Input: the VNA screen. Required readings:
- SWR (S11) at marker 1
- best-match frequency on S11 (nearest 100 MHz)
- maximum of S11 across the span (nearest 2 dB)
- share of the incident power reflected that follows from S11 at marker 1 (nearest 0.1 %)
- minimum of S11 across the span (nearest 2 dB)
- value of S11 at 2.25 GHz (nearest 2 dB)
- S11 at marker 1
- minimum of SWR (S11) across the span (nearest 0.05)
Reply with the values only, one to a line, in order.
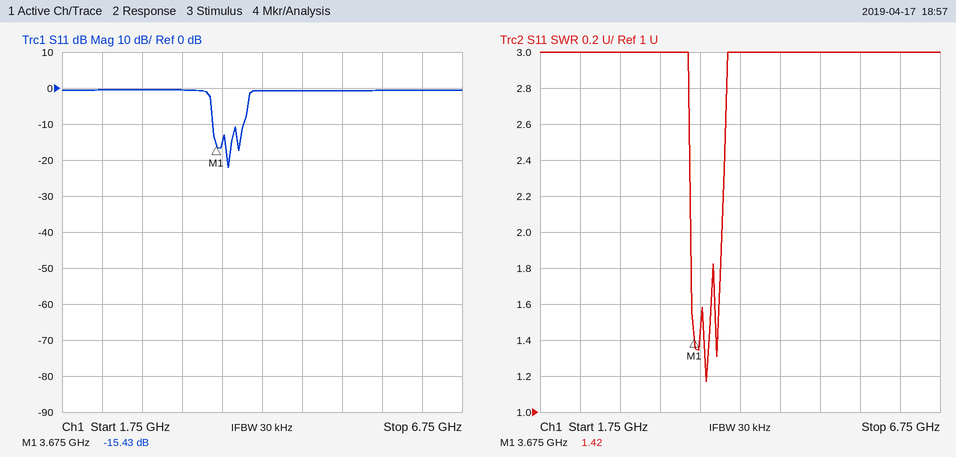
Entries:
1.42
3.8 GHz
0 dB
2.9 %
-22 dB
0 dB
-15.43 dB
1.15
